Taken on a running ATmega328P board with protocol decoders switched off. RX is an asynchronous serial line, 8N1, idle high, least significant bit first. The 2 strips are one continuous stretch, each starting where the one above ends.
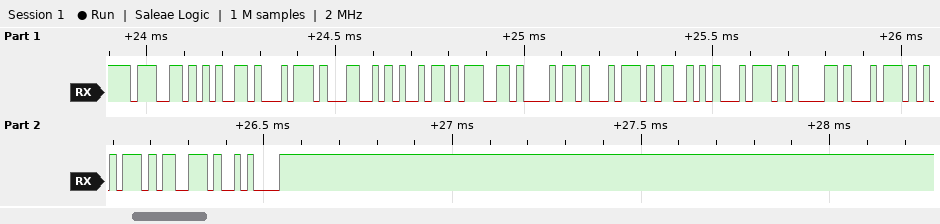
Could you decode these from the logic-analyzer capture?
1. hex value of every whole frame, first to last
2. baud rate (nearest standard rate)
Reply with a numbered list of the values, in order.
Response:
1. 0x67 0x65 0x74 0x4C 0x69 0x67 0x68 0x74 0x53 0x74 0x61 0x74 0x75 0x73 0x0A
2. 57600 baud
